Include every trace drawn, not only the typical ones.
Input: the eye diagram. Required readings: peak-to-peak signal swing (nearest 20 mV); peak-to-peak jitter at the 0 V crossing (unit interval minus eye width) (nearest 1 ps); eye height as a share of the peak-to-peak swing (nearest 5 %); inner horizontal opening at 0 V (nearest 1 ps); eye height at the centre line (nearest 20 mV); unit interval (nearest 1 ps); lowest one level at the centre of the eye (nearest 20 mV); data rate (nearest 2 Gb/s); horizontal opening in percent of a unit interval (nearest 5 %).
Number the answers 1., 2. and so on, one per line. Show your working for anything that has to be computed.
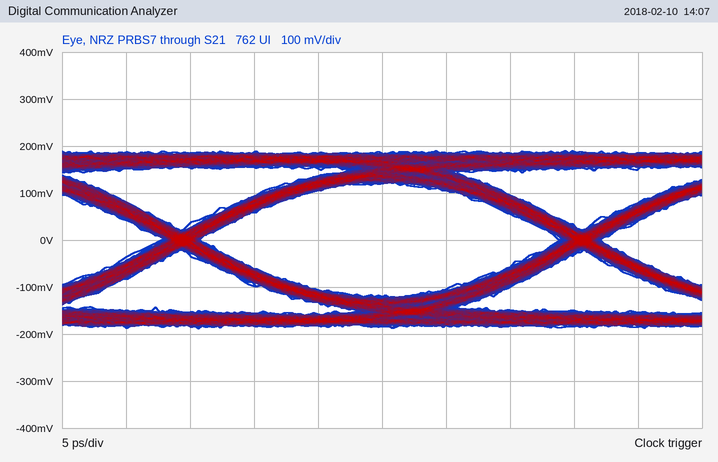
1. 380 mV
2. 3 ps
3. 240 mV / 380 mV ≈ 63.2 %, so 65 % to the nearest 5 %
4. 28 ps
5. 240 mV
6. 31 ps
7. 120 mV
8. 32 Gb/s
9. 28 ps / 31 ps ≈ 90 %
